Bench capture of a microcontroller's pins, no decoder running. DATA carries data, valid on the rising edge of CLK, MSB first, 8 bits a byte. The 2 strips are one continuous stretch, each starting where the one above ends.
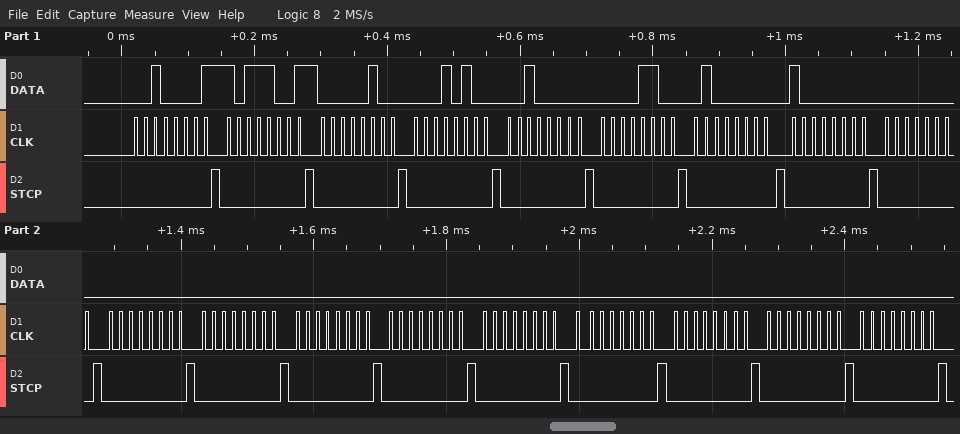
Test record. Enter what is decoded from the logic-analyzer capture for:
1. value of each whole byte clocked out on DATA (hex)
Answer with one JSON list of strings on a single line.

["21 B9 04 14 20 0C 40 80 00 00 00 00 00 00 00 00 00 00"]
